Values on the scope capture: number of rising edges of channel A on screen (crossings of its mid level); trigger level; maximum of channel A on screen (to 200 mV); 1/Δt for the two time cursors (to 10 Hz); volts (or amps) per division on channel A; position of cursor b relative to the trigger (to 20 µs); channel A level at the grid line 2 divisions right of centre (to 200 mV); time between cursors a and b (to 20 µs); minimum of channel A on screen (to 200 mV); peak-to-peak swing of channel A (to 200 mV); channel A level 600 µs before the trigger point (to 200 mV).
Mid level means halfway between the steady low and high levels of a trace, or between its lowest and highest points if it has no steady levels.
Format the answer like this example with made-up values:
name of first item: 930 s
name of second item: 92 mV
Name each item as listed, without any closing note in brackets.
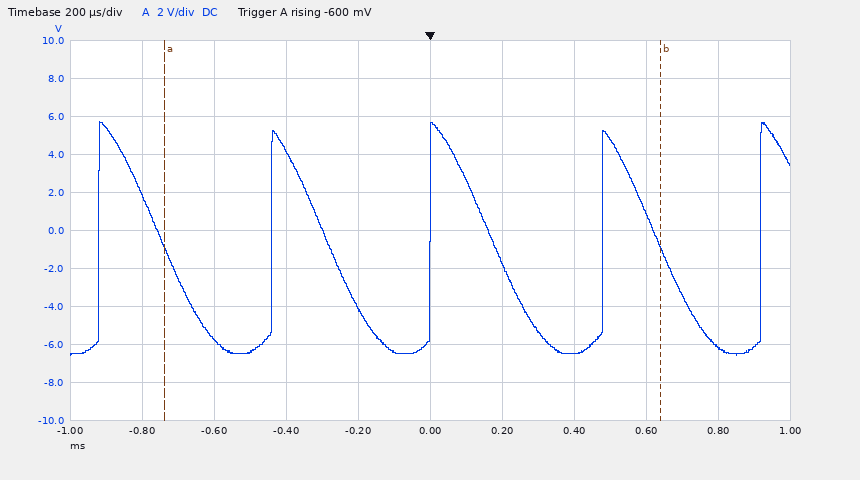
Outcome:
number of rising edges of channel A on screen: 5
trigger level: -600 mV
maximum of channel A on screen: 5.8 V
1/Δt for the two time cursors: 720 Hz
volts (or amps) per division on channel A: 2 V
position of cursor b relative to the trigger: +640 µs
channel A level at the grid line 2 divisions right of centre: -6.4 V
time between cursors a and b: 1.38 ms
minimum of channel A on screen: -6.6 V
peak-to-peak swing of channel A: 12.4 V
channel A level 600 µs before the trigger point: -5.8 V
